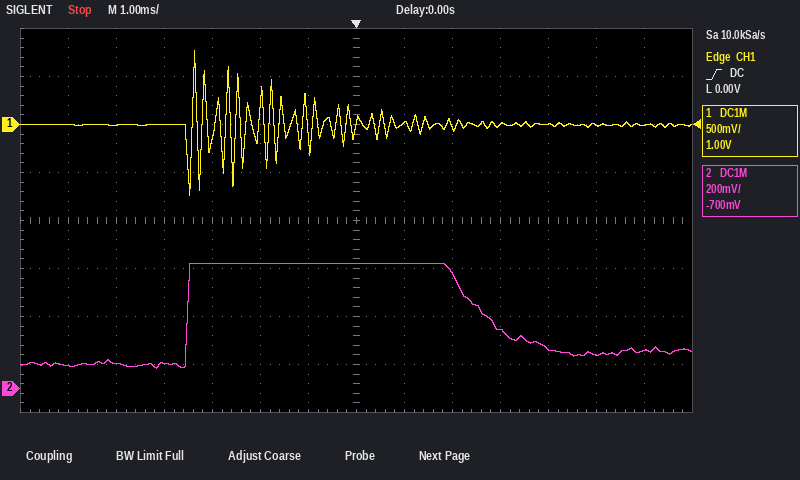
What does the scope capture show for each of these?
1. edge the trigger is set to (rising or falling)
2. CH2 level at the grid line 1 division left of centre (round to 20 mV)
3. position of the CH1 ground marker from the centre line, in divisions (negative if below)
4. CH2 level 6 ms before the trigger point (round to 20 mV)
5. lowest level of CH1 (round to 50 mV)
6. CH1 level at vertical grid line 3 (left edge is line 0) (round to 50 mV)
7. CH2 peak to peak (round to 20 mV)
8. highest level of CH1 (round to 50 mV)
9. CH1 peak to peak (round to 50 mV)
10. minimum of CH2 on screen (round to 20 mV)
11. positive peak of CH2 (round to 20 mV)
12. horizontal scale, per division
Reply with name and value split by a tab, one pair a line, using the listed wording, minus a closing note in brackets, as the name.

edge the trigger is set to	rising
CH2 level at the grid line 1 division left of centre	520 mV
position of the CH1 ground marker from the centre line, in divisions	+2.0 div
CH2 level 6 ms before the trigger point	100 mV
lowest level of CH1	-750 mV
CH1 level at vertical grid line 3 (left edge is line 0)	0 mV
CH2 peak to peak	440 mV
highest level of CH1	750 mV
CH1 peak to peak	1.50 V
minimum of CH2 on screen	80 mV
positive peak of CH2	520 mV
horizontal scale, per division	1 ms
